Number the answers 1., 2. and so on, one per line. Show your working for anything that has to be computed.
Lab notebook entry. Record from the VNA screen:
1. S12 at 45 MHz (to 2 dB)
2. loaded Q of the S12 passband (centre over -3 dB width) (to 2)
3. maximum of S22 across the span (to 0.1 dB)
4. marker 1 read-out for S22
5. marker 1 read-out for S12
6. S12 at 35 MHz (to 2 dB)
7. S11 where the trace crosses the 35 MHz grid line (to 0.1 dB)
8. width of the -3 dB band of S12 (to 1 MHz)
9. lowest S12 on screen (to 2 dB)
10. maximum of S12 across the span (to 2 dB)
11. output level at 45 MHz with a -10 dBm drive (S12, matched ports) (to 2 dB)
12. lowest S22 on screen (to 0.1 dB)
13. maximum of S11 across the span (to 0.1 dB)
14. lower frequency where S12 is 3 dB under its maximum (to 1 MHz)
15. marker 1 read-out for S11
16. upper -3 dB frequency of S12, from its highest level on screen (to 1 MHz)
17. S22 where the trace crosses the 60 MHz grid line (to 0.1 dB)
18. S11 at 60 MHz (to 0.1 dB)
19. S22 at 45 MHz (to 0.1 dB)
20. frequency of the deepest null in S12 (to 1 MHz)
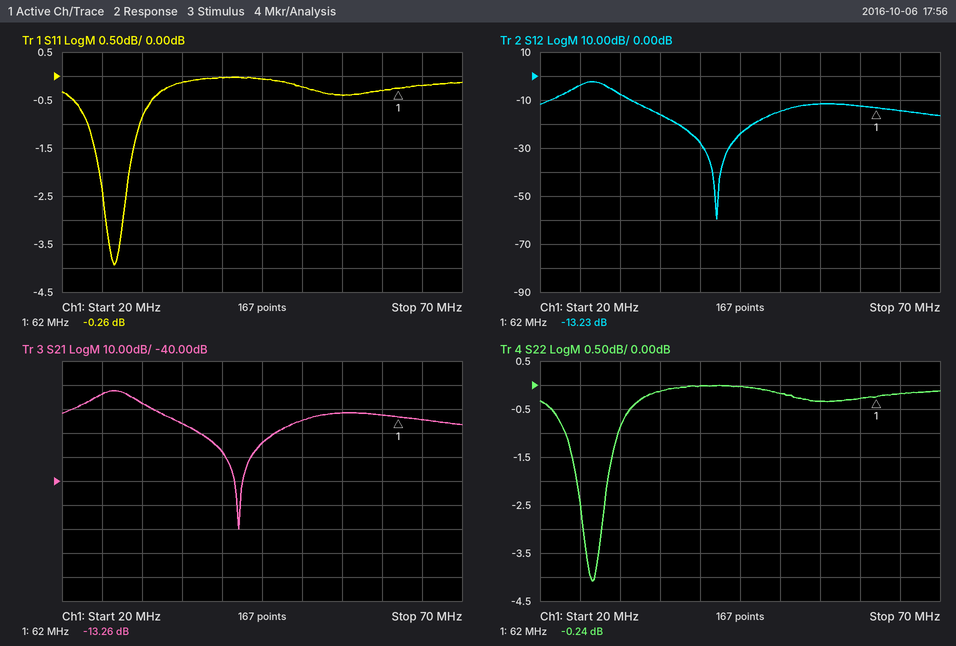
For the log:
1. -24 dB
2. 26.5 MHz / 5 MHz ≈ 5.30, so 6 to the nearest 2
3. 0.0 dB
4. -0.24 dB
5. -13.23 dB
6. -16 dB
7. -0.1 dB
8. 29 MHz − 24 MHz = 5 MHz
9. -60 dB
10. -2 dB
11. -10 dBm + (-24 dB) = -34 dBm
12. -4.1 dB
13. 0.0 dB
14. 24 MHz
15. -0.26 dB
16. 29 MHz
17. -0.3 dB
18. -0.3 dB
19. 0.0 dB
20. 42 MHz
